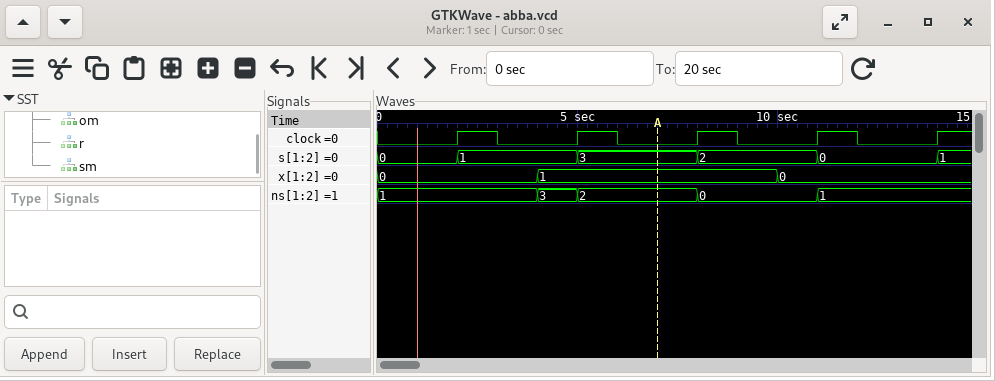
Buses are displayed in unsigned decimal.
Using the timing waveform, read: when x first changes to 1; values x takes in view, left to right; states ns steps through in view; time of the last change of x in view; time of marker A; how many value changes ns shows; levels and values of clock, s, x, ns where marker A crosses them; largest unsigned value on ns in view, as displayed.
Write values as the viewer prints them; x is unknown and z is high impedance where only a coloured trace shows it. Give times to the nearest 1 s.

4 s
0, 1, 0
1, 3, 2, 0, 1
10 s
7 s
4
clock=0, s=3, x=1, ns=2
3
